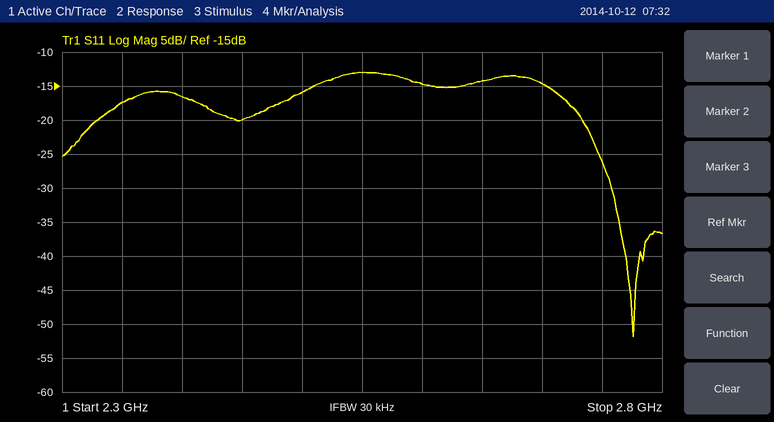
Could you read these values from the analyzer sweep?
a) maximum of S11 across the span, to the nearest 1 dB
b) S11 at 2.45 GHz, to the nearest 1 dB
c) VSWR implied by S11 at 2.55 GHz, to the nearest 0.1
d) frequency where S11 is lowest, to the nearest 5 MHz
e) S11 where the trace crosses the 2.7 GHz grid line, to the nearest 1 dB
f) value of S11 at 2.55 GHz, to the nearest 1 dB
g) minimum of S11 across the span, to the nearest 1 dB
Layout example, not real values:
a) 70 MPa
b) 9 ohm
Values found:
a) -13 dB
b) -20 dB
c) 1.6
d) 2.775 GHz
e) -15 dB
f) -13 dB
g) -52 dB
